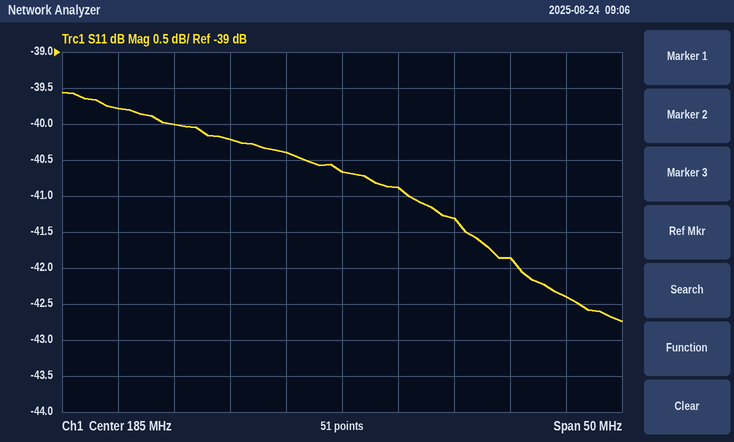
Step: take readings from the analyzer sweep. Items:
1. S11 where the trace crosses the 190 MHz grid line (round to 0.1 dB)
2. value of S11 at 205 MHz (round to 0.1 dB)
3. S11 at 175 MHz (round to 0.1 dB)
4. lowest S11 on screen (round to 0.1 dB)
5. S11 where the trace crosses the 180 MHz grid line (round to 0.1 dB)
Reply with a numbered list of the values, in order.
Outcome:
1. -40.9 dB
2. -42.4 dB
3. -40.2 dB
4. -42.7 dB
5. -40.4 dB
